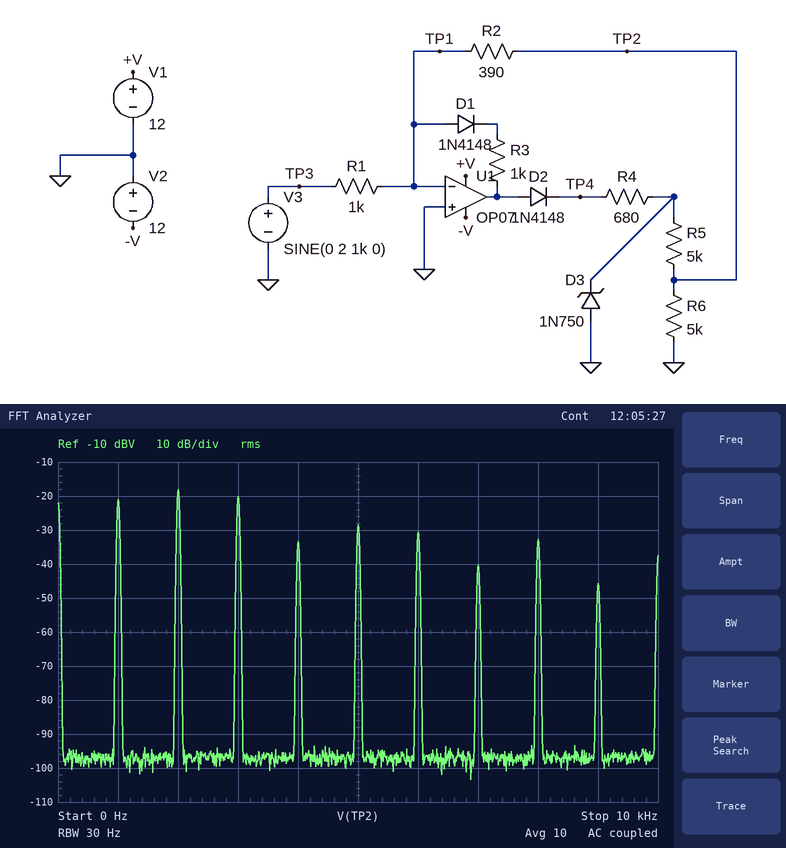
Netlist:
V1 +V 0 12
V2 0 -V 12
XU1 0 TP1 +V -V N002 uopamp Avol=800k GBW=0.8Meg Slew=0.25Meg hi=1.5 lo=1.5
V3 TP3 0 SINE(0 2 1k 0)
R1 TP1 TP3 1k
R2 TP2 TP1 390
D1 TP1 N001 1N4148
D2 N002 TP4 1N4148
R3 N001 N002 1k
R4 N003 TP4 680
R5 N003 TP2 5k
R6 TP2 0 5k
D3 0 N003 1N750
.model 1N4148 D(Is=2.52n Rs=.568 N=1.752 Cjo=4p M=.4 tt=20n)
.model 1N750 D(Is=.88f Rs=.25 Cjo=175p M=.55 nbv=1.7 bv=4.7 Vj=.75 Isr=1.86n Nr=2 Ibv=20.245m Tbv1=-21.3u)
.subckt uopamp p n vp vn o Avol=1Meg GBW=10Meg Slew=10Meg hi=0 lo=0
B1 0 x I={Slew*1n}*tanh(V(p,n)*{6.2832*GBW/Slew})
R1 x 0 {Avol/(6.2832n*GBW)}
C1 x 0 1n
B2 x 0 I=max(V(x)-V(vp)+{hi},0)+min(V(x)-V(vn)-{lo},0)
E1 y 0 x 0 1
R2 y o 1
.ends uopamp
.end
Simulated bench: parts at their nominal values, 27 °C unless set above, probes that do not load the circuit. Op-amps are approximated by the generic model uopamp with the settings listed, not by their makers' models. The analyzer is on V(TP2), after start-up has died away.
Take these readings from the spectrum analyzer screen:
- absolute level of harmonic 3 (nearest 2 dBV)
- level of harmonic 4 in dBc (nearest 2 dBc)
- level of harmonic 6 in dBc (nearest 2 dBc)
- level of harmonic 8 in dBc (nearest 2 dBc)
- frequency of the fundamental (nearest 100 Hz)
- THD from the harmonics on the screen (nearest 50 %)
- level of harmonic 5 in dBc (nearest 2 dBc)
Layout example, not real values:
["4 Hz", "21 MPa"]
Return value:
["-20 dBV", "-12 dBc", "-10 dBc", "-12 dBc", "1.0 kHz", "200 %", "-8 dBc"]
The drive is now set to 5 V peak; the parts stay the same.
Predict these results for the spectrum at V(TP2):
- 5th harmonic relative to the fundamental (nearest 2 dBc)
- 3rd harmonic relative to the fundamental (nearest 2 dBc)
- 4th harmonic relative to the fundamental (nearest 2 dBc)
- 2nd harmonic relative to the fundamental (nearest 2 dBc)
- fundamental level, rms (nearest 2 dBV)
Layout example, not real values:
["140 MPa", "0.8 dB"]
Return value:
["-20 dBc", "-16 dBc", "-18 dBc", "-4 dBc", "-2 dBV"]
